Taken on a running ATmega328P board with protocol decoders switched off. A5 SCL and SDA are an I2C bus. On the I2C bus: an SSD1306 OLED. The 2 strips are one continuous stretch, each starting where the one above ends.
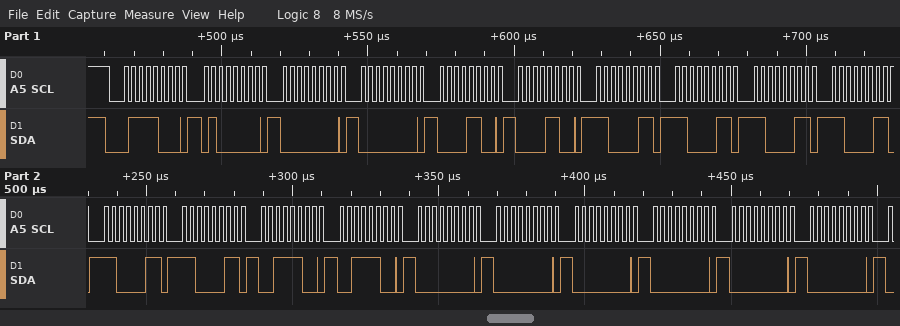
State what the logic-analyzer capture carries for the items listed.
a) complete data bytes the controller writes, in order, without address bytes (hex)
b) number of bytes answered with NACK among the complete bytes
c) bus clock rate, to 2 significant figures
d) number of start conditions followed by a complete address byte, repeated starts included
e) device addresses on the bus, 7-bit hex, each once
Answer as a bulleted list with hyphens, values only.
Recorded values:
- 40 00 00 0C 0C C3 C3 C3 C3 C3 C3 3C 3C 00 00 00 00 00 00
- 0
- 400 kHz
- 1
- 0x3C
